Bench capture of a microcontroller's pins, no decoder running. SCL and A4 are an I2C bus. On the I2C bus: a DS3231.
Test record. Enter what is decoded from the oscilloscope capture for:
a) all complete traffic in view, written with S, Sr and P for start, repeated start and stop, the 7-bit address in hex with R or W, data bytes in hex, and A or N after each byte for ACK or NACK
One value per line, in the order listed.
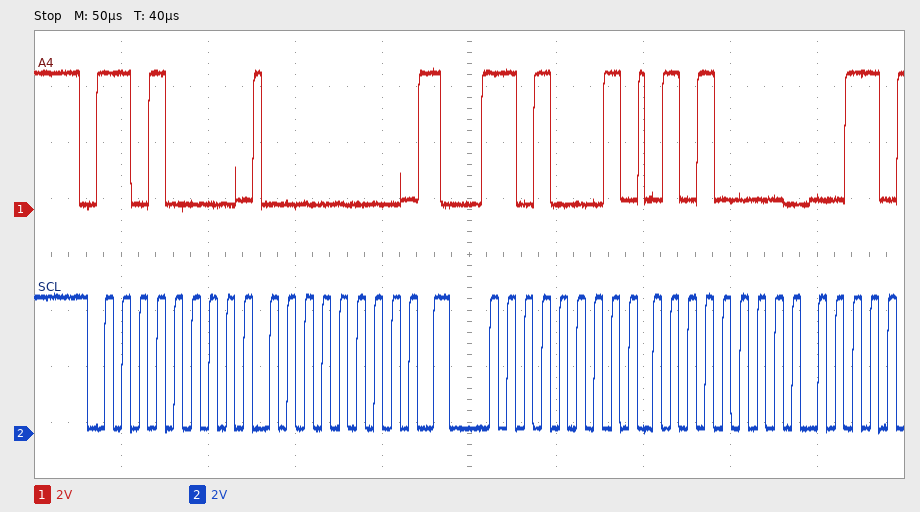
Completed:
S 68W A 00 A Sr 68R A 50 A
